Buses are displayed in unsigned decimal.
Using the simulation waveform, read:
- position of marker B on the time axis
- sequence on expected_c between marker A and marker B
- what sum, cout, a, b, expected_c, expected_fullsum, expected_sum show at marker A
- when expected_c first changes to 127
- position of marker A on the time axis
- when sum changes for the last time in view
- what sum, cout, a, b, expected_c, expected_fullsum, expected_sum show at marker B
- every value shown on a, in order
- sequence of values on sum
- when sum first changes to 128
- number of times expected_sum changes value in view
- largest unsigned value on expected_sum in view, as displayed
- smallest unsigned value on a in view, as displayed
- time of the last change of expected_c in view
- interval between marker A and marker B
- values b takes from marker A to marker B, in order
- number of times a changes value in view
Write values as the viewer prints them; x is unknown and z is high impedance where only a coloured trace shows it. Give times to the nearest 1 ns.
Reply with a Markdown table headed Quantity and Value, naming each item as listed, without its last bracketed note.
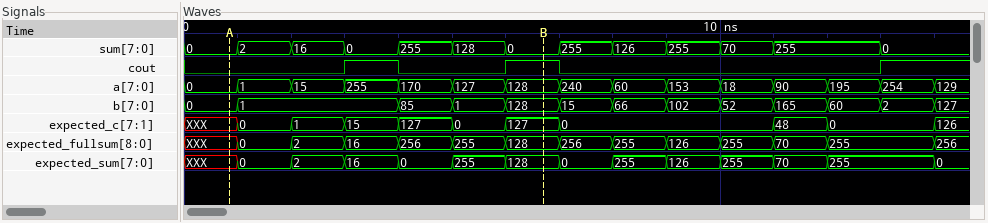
| Quantity | Value |
|---|---|
| position of marker B on the time axis | 7 ns |
| sequence on expected_c between marker A and marker B | XXX, 0, 1, 15, 127, 0, 127 |
| what sum, cout, a, b, expected_c, expected_fullsum, expected_sum show at marker A | sum=0, cout=0, a=0, b=0, expected_c=XXX, expected_fullsum=XXX, expected_sum=XXX |
| when expected_c first changes to 127 | 4 ns |
| position of marker A on the time axis | 1 ns |
| when sum changes for the last time in view | 13 ns |
| what sum, cout, a, b, expected_c, expected_fullsum, expected_sum show at marker B | sum=0, cout=1, a=128, b=128, expected_c=127, expected_fullsum=128, expected_sum=128 |
| every value shown on a, in order | 0, 1, 15, 255, 170, 127, 128, 240, 60, 153, 18, 90, 195, 254, 129 |
| sequence of values on sum | 0, 2, 16, 0, 255, 128, 0, 255, 126, 255, 70, 255, 0 |
| when sum first changes to 128 | 5 ns |
| number of times expected_sum changes value in view | 13 |
| largest unsigned value on expected_sum in view, as displayed | 255 |
| smallest unsigned value on a in view, as displayed | 0 |
| time of the last change of expected_c in view | 14 ns |
| interval between marker A and marker B | 6 ns |
| values b takes from marker A to marker B, in order | 0, 1, 85, 1, 128 |
| number of times a changes value in view | 14 |
